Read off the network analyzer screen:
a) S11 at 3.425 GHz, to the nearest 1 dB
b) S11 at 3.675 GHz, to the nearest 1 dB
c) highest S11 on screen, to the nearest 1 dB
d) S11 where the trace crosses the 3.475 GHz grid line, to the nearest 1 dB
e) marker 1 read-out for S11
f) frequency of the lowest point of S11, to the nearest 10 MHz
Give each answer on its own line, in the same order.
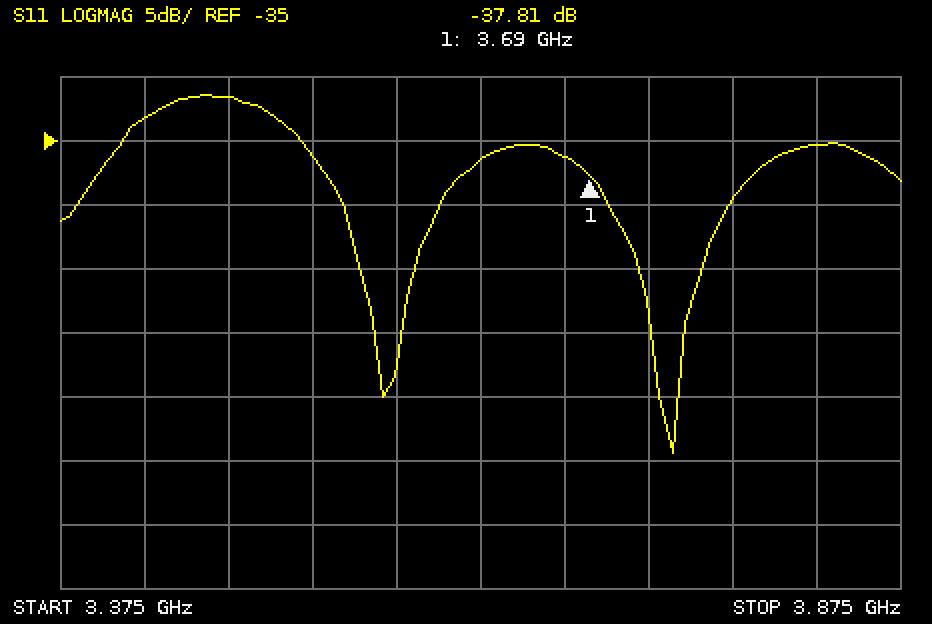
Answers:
-33 dB
-36 dB
-31 dB
-32 dB
-37.81 dB
3.74 GHz
